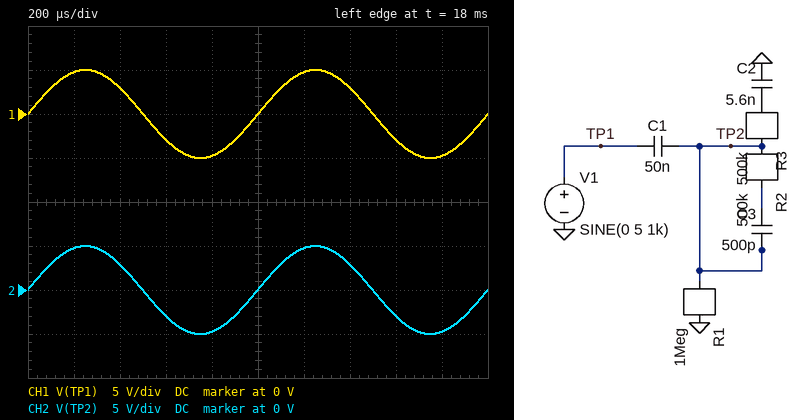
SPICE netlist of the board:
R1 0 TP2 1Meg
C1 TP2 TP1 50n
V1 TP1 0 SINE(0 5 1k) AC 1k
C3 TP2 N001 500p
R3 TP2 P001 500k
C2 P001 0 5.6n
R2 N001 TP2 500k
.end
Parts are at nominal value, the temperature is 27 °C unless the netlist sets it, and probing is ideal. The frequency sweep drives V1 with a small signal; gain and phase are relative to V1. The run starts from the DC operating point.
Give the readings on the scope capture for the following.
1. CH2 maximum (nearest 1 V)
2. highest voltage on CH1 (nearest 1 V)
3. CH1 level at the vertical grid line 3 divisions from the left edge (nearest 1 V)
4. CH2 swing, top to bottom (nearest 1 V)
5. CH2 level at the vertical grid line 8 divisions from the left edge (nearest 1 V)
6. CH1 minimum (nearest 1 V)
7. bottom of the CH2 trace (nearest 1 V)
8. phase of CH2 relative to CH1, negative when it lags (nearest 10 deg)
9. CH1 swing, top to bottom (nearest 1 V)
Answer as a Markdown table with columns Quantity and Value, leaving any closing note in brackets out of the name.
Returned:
| Quantity | Value |
|---|---|
| CH2 maximum | 5 V |
| highest voltage on CH1 | 5 V |
| CH1 level at the vertical grid line 3 divisions from the left edge | -3 V |
| CH2 swing, top to bottom | 10 V |
| CH2 level at the vertical grid line 8 divisions from the left edge | -3 V |
| CH1 minimum | -5 V |
| bottom of the CH2 trace | -5 V |
| phase of CH2 relative to CH1, negative when it lags | 0 deg |
| CH1 swing, top to bottom | 10 V |
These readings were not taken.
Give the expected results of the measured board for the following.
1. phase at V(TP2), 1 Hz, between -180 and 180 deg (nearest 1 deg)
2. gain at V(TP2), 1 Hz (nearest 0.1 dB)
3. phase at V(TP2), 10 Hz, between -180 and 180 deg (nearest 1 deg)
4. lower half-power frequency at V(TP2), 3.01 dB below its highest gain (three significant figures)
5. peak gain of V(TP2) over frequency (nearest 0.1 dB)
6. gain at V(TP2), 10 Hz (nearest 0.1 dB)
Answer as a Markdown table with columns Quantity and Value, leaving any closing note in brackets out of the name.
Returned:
| Quantity | Value |
|---|---|
| phase at V(TP2), 1 Hz, between -180 and 180 deg | 71 deg |
| gain at V(TP2), 1 Hz | -10.6 dB |
| phase at V(TP2), 10 Hz, between -180 and 180 deg | 17 deg |
| lower half-power frequency at V(TP2), 3.01 dB below its highest gain | 3.67 Hz |
| peak gain of V(TP2) over frequency | 0 dB |
| gain at V(TP2), 10 Hz | -1.3 dB |
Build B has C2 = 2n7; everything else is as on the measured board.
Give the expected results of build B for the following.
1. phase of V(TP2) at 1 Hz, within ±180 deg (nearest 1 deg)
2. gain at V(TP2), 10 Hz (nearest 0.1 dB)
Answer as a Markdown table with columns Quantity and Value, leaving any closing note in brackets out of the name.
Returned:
| Quantity | Value |
|---|---|
| phase of V(TP2) at 1 Hz, within ±180 deg | 72 deg |
| gain at V(TP2), 10 Hz | -0.8 dB |
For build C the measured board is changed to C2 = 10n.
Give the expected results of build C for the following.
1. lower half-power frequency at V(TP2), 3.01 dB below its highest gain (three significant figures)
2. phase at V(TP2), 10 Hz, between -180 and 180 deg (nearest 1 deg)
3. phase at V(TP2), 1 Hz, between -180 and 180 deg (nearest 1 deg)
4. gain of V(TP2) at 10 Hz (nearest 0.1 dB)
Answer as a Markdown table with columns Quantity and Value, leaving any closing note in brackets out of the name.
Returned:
| Quantity | Value |
|---|---|
| lower half-power frequency at V(TP2), 3.01 dB below its highest gain | 4.38 Hz |
| phase at V(TP2), 10 Hz, between -180 and 180 deg | 18 deg |
| phase at V(TP2), 1 Hz, between -180 and 180 deg | 69 deg |
| gain of V(TP2) at 10 Hz | -1.9 dB |
